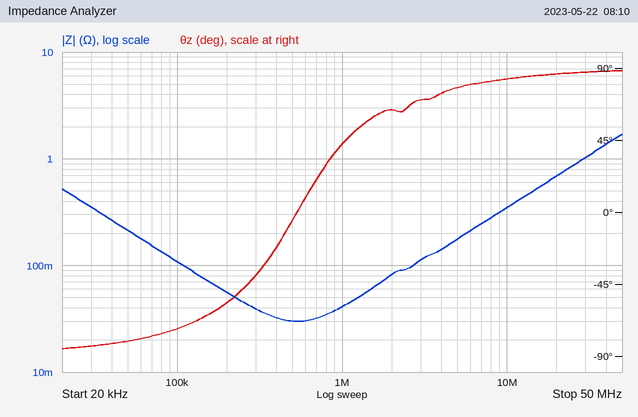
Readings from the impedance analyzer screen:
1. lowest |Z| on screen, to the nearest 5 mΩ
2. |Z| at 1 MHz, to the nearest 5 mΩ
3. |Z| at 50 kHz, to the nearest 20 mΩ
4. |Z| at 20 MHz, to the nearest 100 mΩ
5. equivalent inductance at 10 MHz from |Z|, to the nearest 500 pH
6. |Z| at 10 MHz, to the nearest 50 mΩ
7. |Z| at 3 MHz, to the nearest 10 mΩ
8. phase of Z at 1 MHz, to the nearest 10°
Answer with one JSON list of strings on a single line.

["30 mΩ", "40 mΩ", "220 mΩ", "700 mΩ", "5.5 nH", "350 mΩ", "110 mΩ", "40°"]
